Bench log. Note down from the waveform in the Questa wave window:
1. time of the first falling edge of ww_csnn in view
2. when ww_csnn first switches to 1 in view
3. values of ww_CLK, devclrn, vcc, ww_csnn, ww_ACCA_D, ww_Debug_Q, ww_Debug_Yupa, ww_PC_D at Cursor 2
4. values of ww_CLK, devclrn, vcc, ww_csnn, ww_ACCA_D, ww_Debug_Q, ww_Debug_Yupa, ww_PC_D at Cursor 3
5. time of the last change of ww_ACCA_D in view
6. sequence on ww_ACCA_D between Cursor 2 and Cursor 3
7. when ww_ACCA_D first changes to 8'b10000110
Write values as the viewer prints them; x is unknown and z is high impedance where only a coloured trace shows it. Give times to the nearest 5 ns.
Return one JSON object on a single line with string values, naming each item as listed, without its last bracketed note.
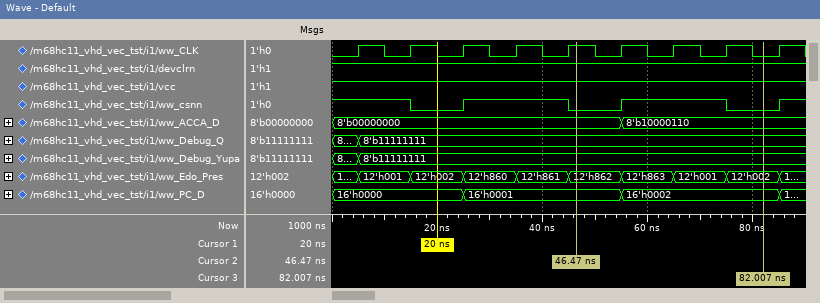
{"time of the first falling edge of ww_csnn in view": "15 ns", "when ww_csnn first switches to 1 in view": "25 ns", "values of ww_CLK, devclrn, vcc, ww_csnn, ww_ACCA_D, ww_Debug_Q, ww_Debug_Yupa, ww_PC_D at Cursor 2": "ww_CLK=1, devclrn=1, vcc=1, ww_csnn=0, ww_ACCA_D=8'b00000000, ww_Debug_Q=8'b11111111, ww_Debug_Yupa=8'b11111111, ww_PC_D=16'h0001", "values of ww_CLK, devclrn, vcc, ww_csnn, ww_ACCA_D, ww_Debug_Q, ww_Debug_Yupa, ww_PC_D at Cursor 3": "ww_CLK=0, devclrn=1, vcc=1, ww_csnn=0, ww_ACCA_D=8'b10000110, ww_Debug_Q=8'b11111111, ww_Debug_Yupa=8'b11111111, ww_PC_D=16'h0002", "time of the last change of ww_ACCA_D in view": "55 ns", "sequence on ww_ACCA_D between Cursor 2 and Cursor 3": "8'b00000000, 8'b10000110", "when ww_ACCA_D first changes to 8'b10000110": "55 ns"}
